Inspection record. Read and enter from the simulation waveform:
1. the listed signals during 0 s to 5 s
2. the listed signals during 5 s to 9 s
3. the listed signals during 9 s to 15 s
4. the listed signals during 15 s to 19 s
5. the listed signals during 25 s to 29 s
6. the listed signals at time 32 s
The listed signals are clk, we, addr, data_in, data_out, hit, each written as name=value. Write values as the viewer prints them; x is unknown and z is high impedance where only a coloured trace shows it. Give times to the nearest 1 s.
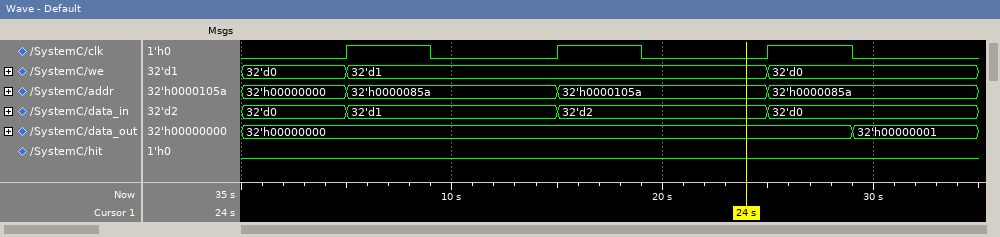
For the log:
clk=0, we=32'd0, addr=32'h00000000, data_in=32'd0, data_out=32'h00000000, hit=0
clk=1, we=32'd1, addr=32'h0000085a, data_in=32'd1, data_out=32'h00000000, hit=0
clk=0, we=32'd1, addr=32'h0000085a, data_in=32'd1, data_out=32'h00000000, hit=0
clk=1, we=32'd1, addr=32'h0000105a, data_in=32'd2, data_out=32'h00000000, hit=0
clk=1, we=32'd0, addr=32'h0000085a, data_in=32'd0, data_out=32'h00000000, hit=0
clk=0, we=32'd0, addr=32'h0000085a, data_in=32'd0, data_out=32'h00000001, hit=0
